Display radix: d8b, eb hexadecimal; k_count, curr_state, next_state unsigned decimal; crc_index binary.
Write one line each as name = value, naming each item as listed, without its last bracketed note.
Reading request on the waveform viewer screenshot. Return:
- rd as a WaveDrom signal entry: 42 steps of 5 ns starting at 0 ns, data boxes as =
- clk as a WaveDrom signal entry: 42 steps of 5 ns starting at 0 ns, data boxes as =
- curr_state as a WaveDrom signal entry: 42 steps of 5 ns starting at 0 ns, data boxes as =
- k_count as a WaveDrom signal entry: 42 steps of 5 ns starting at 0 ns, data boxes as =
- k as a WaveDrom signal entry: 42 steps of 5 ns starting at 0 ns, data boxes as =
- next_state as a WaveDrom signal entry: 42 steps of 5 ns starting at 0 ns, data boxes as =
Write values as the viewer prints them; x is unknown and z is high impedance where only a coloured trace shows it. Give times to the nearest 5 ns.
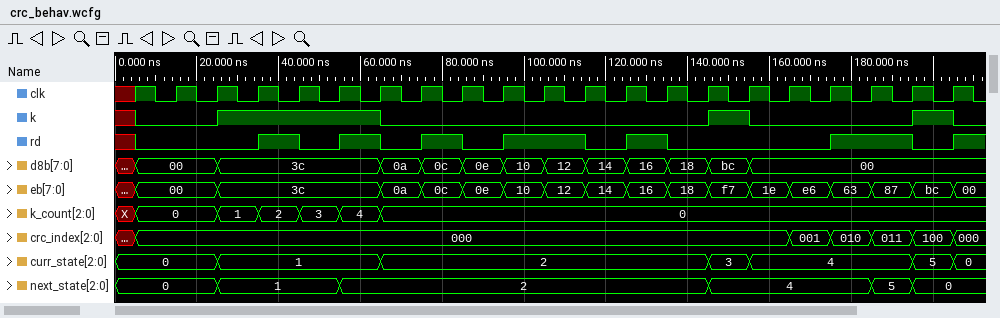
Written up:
rd as a WaveDrom signal entry: 42 steps of 5 ns starting at 0 ns, data boxes as = = {name: 'rd', wave: 'x0.....1.0.1.0.1.0.1...0.1.0.......1...0.1'}
clk as a WaveDrom signal entry: 42 steps of 5 ns starting at 0 ns, data boxes as = = {name: 'clk', wave: 'x10101010101010101010101010101010101010101'}
curr_state as a WaveDrom signal entry: 42 steps of 5 ns starting at 0 ns, data boxes as = = {name: 'curr_state', wave: '=....=.......=...............=.=.......=.=', data: '0 1 2 3 4 5 0'}
k_count as a WaveDrom signal entry: 42 steps of 5 ns starting at 0 ns, data boxes as = = {name: 'k_count', wave: 'x=...=.=.=.=.=............................', data: '0 1 2 3 4 0'}
k as a WaveDrom signal entry: 42 steps of 5 ns starting at 0 ns, data boxes as = = {name: 'k', wave: 'x0...1.......0...............1.0.......1.0'}
next_state as a WaveDrom signal entry: 42 steps of 5 ns starting at 0 ns, data boxes as = = {name: 'next_state', wave: '=....=.....=.................=.......=.=..', data: '0 1 2 4 5 0'}
